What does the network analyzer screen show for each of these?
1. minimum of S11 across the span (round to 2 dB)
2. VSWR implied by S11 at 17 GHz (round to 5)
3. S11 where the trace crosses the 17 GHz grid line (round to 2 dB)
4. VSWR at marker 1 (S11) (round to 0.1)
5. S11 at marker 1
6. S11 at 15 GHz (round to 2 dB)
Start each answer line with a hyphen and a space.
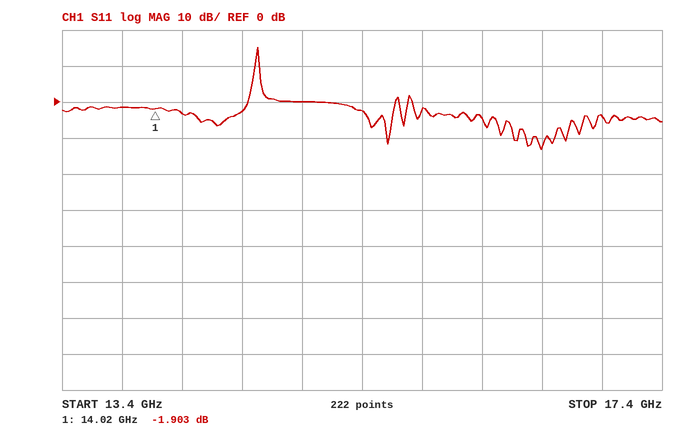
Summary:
- -14 dB
- 5
- -4 dB
- 9.2
- -1.903 dB
- 0 dB
